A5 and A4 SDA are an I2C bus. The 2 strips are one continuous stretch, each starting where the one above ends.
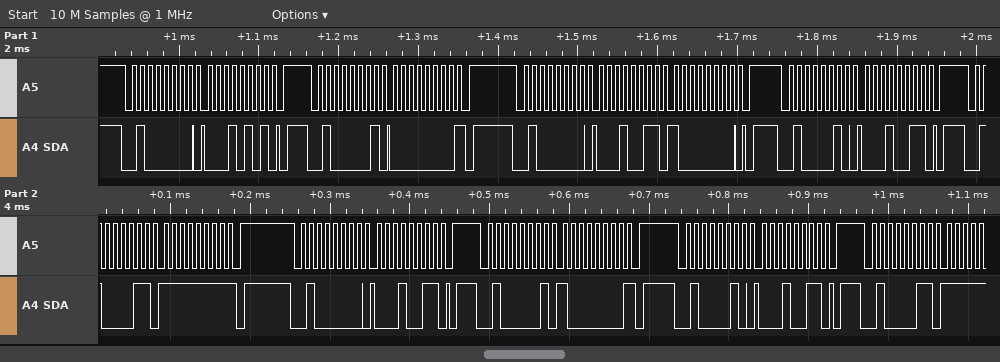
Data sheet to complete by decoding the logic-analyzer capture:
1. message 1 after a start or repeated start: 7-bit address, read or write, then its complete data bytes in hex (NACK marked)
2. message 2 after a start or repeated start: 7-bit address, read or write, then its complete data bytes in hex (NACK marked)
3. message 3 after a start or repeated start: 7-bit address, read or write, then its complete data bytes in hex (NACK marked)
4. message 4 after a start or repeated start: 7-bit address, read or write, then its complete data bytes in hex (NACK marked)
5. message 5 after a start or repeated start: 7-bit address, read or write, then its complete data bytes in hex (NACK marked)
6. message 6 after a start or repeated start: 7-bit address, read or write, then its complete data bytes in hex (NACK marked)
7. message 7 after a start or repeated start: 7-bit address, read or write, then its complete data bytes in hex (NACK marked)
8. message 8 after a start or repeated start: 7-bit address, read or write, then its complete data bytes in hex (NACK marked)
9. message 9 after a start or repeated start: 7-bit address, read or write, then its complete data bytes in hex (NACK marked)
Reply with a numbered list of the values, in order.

1. 0x20 write: 15
2. 0x20 read: 00 NACK
3. 0x20 write: 13 80
4. 0x21 write: 13
5. 0x21 read: FF NACK
6. 0x20 write: 13
7. 0x20 read: 80 NACK
8. 0x21 write: 13
9. 0x21 read
